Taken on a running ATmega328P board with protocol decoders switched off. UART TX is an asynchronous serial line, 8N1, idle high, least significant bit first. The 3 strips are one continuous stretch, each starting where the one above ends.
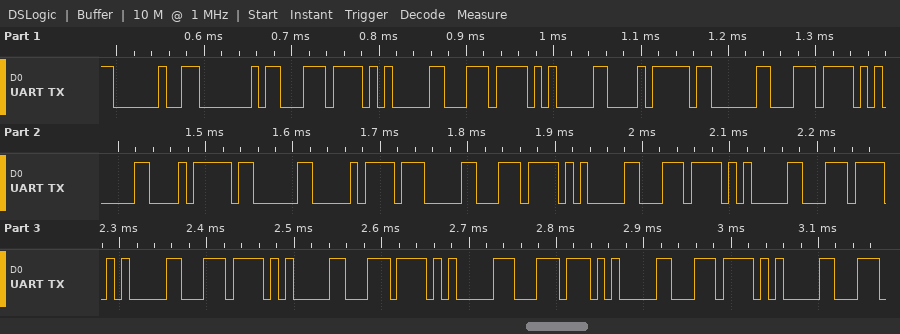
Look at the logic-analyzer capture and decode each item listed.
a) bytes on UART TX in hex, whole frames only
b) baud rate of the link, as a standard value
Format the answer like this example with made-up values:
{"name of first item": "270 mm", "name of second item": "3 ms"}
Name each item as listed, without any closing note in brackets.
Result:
{"bytes on UART TX in hex, whole frames only": "20 40 DC 05 DC 05 E8 03 DC 05 E8 03 D0 07 DC 05 DC 05 DC 05 DC 05 DC 05 DC 05 DC 05", "baud rate of the link, as a standard value": "115200 baud"}
